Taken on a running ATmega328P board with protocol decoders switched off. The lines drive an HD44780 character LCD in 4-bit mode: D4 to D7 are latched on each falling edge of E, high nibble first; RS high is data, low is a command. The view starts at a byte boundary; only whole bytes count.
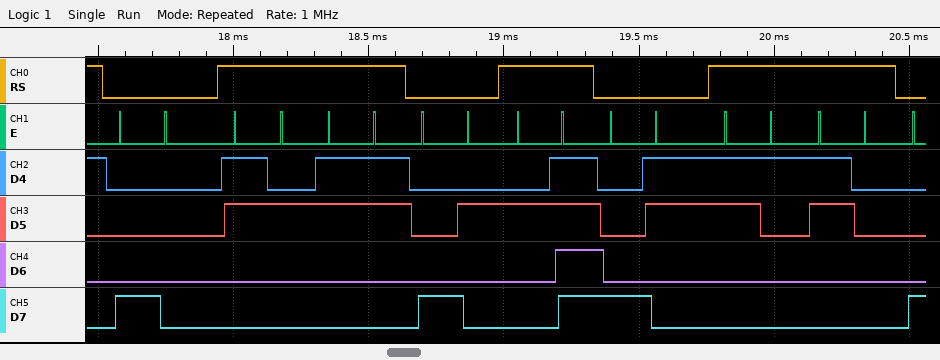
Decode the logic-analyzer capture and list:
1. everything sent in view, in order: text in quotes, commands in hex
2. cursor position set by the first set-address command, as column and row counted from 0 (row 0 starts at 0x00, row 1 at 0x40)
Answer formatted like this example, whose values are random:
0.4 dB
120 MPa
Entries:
0x80 "23" 0x82 "/" 0x83 "10"
column 0, row 0
